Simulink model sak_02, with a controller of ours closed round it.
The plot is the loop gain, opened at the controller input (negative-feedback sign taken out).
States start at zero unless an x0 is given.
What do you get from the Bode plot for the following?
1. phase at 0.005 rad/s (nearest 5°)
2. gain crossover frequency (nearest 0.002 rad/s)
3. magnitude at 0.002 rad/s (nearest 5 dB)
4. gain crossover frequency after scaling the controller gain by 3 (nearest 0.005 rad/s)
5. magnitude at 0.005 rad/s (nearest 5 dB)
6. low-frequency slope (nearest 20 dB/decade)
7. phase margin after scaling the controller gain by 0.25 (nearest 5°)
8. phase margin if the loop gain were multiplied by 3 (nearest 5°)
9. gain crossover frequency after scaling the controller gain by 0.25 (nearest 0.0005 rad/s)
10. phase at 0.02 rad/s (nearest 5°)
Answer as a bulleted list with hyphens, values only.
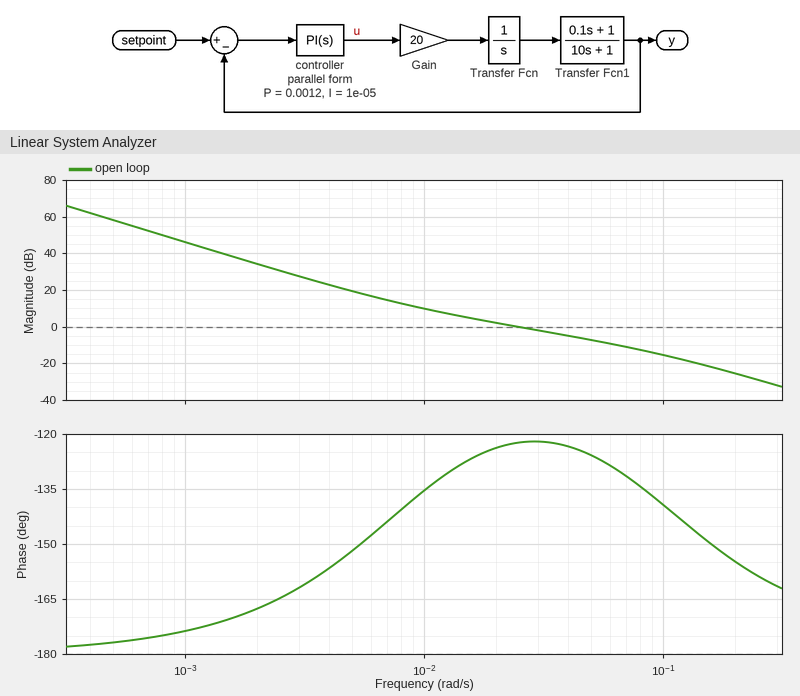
- -150°
- 0.024 rad/s
- 35 dB
- 0.060 rad/s
- 20 dB
- -40 dB/decade
- 40°
- 50°
- 0.0085 rad/s
- -125°
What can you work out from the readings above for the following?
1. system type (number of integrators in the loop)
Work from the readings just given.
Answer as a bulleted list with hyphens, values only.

- 2
